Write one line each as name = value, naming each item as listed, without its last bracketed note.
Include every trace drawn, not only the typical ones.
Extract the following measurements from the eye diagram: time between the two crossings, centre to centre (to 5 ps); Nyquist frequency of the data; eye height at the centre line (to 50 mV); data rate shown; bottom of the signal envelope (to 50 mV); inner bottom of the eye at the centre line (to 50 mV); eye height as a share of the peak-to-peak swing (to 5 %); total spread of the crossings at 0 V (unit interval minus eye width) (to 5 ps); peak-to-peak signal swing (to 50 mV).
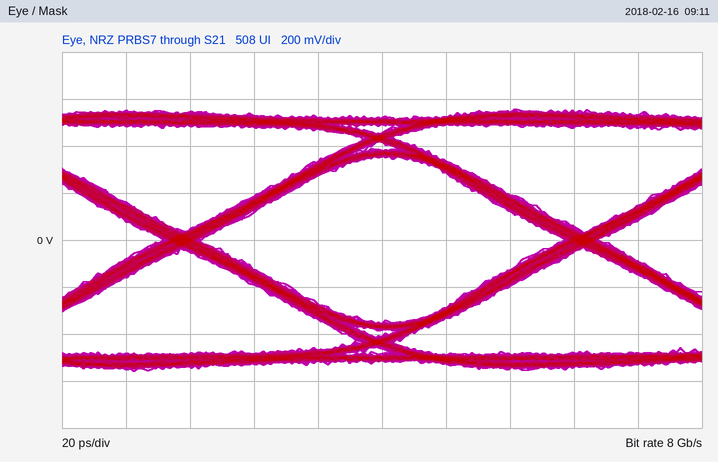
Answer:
time between the two crossings, centre to centre = 125 ps
Nyquist frequency of the data = 4 GHz
eye height at the centre line = 700 mV
data rate shown = 8 Gb/s
bottom of the signal envelope = -550 mV
inner bottom of the eye at the centre line = -350 mV
eye height as a share of the peak-to-peak swing = 65 %
total spread of the crossings at 0 V (unit interval minus eye width) = 10 ps
peak-to-peak signal swing = 1.10 V
